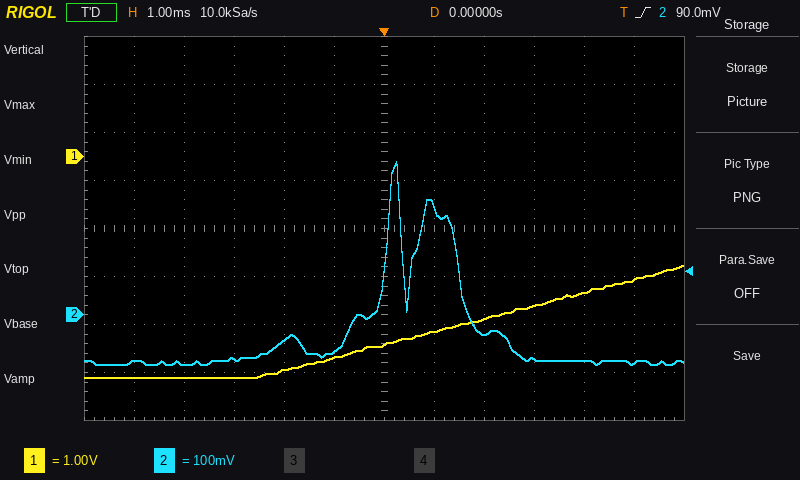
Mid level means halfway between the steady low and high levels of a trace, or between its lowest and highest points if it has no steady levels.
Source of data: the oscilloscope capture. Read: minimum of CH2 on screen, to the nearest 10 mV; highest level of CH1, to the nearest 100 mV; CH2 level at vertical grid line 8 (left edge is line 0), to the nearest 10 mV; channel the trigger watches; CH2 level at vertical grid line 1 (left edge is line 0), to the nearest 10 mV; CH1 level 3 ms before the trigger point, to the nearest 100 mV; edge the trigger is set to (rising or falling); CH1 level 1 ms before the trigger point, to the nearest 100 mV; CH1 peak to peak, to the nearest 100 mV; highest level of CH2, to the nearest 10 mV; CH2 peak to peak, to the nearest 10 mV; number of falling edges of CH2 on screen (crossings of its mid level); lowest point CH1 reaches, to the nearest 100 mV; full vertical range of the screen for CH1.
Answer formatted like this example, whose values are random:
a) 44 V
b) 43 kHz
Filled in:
a) -100 mV
b) -2.3 V
c) -40 mV
d) CH2
e) -100 mV
f) -4.6 V
g) rising
h) -4.2 V
i) 2.3 V
j) 320 mV
k) 420 mV
l) 2
m) -4.6 V
n) 8 V
